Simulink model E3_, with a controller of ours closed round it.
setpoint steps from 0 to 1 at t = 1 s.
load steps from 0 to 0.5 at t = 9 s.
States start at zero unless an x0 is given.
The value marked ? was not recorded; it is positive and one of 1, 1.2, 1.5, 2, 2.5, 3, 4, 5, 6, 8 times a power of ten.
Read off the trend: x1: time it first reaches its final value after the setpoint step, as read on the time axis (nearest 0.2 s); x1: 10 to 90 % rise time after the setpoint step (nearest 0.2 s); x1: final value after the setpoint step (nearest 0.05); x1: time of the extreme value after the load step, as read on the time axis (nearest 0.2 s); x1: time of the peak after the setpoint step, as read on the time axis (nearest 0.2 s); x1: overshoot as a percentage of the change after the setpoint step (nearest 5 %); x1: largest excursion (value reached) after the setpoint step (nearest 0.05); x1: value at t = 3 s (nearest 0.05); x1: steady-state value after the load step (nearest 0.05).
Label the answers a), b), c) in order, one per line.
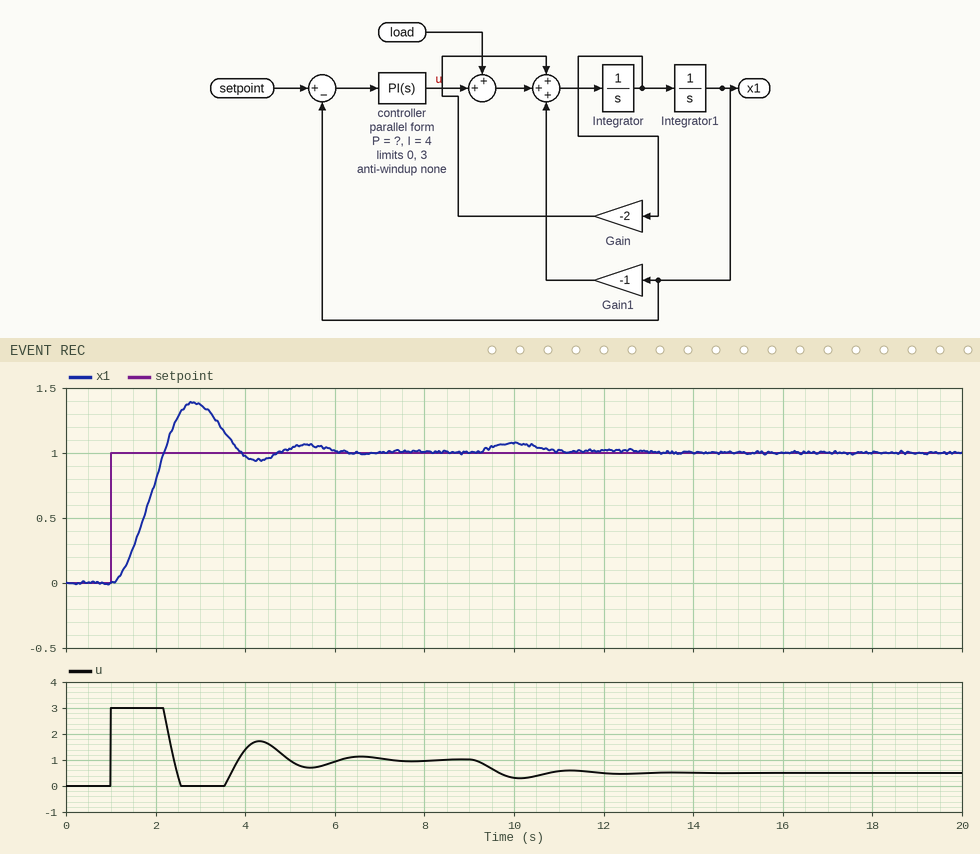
a) 2.2 s
b) 0.8 s
c) 1.00
d) 10.0 s
e) 2.8 s
f) 40 %
g) 1.40
h) 1.35
i) 1.00
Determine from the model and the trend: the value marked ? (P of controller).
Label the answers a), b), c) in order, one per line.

a) 8
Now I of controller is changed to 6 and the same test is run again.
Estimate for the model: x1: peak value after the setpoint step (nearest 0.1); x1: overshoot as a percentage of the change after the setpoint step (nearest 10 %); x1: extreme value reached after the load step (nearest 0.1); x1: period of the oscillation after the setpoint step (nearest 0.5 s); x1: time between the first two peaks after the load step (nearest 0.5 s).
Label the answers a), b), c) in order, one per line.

a) 1.5
b) 50 %
c) 1.1
d) 3.0 s
e) 2.5 s
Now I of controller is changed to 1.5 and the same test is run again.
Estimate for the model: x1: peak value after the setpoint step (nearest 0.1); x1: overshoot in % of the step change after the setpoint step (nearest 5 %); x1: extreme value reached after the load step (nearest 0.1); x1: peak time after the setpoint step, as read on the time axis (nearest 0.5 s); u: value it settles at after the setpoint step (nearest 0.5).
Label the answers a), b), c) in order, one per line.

a) 1.2
b) 20 %
c) 1.1
d) 2.5 s
e) 1.0
